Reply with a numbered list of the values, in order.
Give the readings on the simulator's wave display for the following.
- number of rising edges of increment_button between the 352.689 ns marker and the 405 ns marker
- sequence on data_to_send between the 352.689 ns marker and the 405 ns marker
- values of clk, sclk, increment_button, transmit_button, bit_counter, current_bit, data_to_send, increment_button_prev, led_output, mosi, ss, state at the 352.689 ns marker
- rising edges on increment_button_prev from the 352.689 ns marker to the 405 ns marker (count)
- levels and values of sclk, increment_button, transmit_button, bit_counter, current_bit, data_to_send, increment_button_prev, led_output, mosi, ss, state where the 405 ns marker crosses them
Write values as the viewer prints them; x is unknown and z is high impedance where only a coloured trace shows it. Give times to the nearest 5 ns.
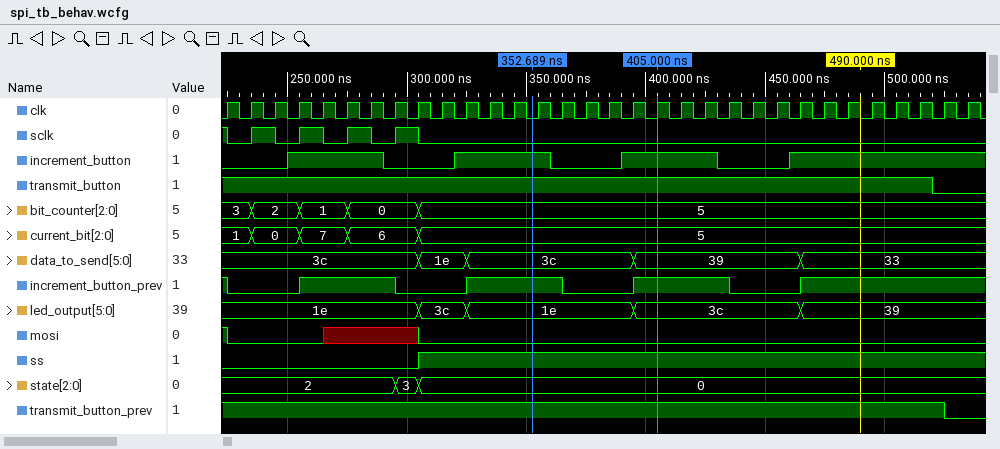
1. 1
2. 3c, 39
3. clk=0, sclk=0, increment_button=1, transmit_button=1, bit_counter=5, current_bit=5, data_to_send=3c, increment_button_prev=1, led_output=1e, mosi=0, ss=1, state=0
4. 1
5. sclk=0, increment_button=1, transmit_button=1, bit_counter=5, current_bit=5, data_to_send=39, increment_button_prev=1, led_output=3c, mosi=0, ss=1, state=0
